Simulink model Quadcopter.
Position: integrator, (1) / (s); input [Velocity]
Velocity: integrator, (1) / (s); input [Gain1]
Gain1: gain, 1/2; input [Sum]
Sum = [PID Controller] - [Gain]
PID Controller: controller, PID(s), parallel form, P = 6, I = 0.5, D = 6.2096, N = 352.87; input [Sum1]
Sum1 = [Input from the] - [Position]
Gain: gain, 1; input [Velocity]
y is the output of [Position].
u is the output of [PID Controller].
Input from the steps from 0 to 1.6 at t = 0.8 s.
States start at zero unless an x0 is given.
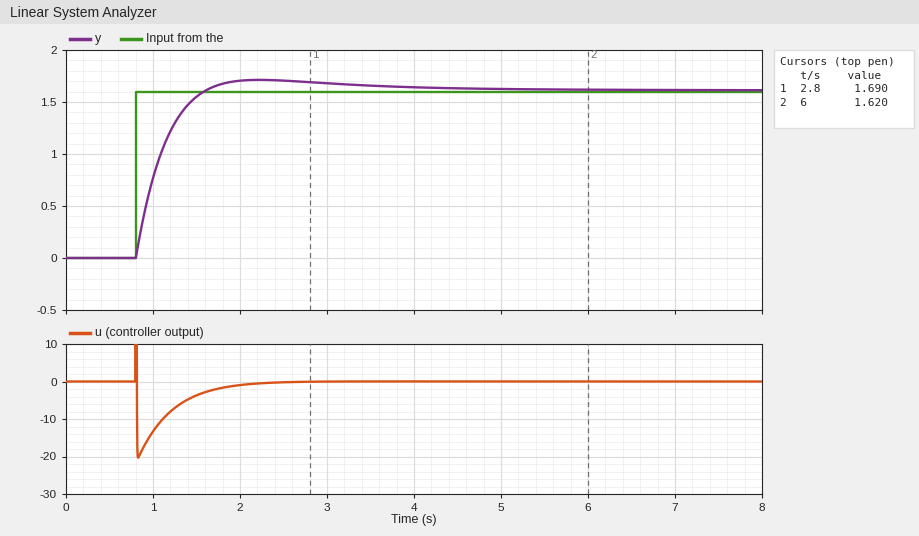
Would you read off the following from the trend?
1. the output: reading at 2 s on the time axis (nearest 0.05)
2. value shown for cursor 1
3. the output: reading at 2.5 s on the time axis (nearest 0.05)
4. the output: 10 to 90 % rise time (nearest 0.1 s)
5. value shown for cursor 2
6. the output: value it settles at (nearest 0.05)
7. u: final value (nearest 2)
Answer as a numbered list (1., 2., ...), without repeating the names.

1. 1.70
2. 1.690
3. 1.70
4. 0.5 s
5. 1.620
6. 1.60
7. 0
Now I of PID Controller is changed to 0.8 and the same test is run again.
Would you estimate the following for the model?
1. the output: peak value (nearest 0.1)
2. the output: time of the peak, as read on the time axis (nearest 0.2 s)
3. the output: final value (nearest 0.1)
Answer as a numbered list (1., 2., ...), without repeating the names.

1. 1.7
2. 2.2 s
3. 1.6
